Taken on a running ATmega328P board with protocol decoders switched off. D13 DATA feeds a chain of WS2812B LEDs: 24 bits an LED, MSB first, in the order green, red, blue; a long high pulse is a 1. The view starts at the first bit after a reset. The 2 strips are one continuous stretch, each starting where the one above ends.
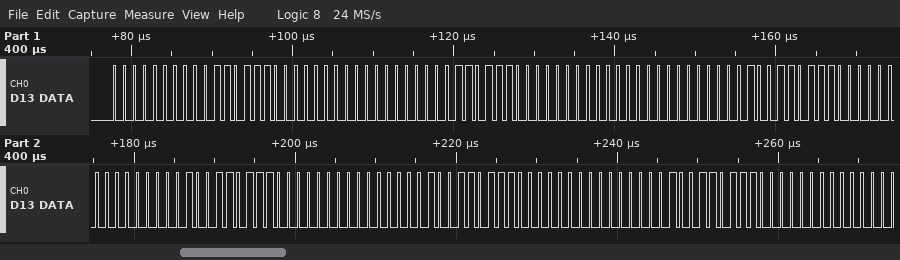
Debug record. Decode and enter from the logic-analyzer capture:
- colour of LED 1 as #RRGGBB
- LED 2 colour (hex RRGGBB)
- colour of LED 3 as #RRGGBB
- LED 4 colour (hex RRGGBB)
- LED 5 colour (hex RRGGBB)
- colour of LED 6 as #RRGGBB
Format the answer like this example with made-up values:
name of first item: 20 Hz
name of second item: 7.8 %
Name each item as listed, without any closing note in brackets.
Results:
colour of LED 1 as #RRGGBB: #370000
LED 2 colour: #370000
colour of LED 3 as #RRGGBB: #010037
LED 4 colour: #010037
LED 5 colour: #010037
colour of LED 6 as #RRGGBB: #010037
